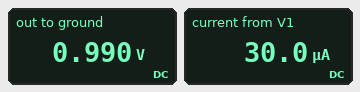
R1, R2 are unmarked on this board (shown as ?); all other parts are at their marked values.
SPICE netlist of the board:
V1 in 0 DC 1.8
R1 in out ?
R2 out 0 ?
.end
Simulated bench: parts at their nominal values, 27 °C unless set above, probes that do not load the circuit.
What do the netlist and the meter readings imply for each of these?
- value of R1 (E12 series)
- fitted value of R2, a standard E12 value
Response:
27 kΩ
33 kΩ
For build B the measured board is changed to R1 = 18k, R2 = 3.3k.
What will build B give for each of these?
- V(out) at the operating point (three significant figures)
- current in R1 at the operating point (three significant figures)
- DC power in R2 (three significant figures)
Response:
279 mV
84.5 µA
23.6 µW
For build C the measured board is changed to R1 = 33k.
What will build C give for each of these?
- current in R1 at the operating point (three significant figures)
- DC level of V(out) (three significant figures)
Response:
27.3 µA
900 mV
